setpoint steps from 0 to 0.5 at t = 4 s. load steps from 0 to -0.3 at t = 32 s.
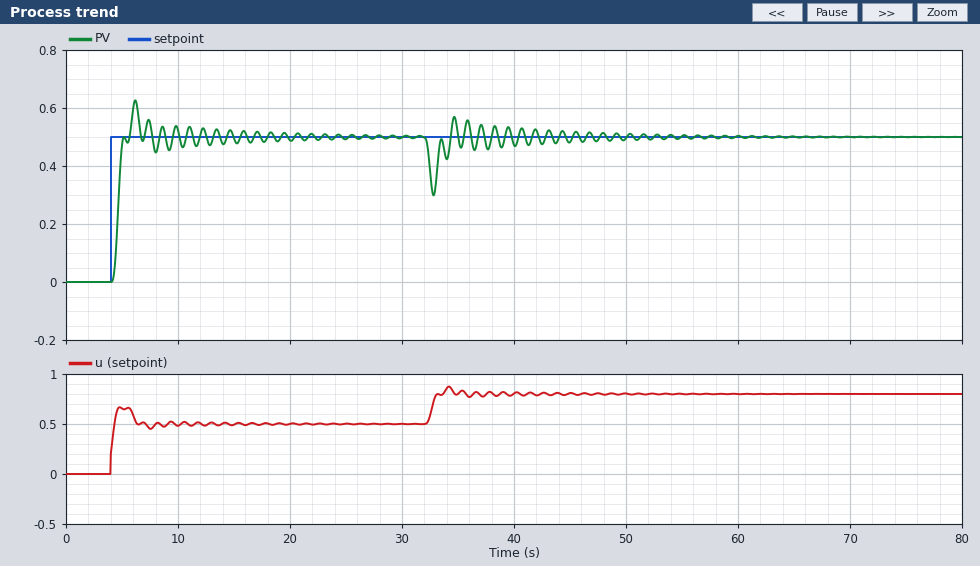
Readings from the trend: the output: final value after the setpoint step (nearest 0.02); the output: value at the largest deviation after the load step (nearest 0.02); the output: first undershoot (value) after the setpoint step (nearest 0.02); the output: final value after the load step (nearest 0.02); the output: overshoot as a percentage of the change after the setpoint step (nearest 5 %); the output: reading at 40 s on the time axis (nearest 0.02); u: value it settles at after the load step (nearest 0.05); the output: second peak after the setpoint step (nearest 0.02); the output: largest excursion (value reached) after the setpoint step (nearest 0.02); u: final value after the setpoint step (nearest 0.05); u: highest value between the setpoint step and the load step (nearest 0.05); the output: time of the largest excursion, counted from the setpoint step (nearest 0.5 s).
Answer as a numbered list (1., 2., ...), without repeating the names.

1. 0.50
2. 0.30
3. 0.48
4. 0.50
5. 25 %
6. 0.48
7. 0.80
8. 0.56
9. 0.62
10. 0.50
11. 0.65
12. 2.0 s
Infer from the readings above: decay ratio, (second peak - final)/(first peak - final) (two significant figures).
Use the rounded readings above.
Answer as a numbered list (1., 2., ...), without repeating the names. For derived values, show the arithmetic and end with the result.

1. (0.56 - 0.5) / (0.62 - 0.5) = 0.50
